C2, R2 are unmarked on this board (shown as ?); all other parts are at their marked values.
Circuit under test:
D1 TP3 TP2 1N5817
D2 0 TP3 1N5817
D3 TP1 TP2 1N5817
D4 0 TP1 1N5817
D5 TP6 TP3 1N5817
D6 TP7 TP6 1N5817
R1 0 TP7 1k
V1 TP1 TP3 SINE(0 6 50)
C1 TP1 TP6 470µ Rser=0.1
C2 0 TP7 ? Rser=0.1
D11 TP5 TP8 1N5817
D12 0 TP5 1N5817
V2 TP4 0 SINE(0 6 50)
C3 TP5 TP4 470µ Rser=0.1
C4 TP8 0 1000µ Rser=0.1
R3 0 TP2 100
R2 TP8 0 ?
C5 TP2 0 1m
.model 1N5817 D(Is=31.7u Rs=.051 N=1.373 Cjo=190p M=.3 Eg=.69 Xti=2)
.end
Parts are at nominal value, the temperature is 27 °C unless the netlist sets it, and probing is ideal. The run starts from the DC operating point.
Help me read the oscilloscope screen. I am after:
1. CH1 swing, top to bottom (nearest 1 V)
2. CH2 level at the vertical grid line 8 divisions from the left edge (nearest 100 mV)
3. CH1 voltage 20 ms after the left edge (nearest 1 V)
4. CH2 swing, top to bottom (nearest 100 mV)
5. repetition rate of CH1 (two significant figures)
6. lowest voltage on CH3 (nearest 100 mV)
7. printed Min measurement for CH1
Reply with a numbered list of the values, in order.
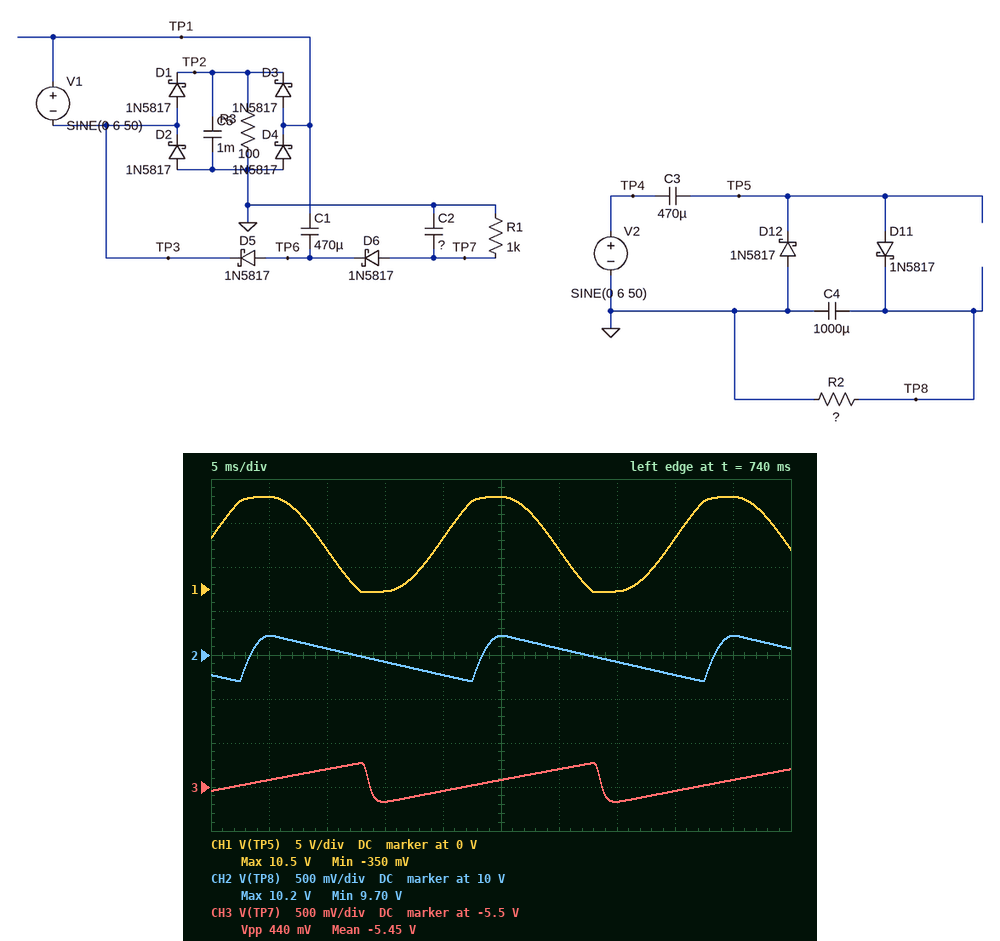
1. 11 V
2. 9.8 V
3. 6 V
4. 500 mV
5. 50 Hz
6. -5.7 V
7. -350 mV
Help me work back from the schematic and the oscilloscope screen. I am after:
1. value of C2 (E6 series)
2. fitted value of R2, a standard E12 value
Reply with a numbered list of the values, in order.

1. 220 µF
2. 330 Ω
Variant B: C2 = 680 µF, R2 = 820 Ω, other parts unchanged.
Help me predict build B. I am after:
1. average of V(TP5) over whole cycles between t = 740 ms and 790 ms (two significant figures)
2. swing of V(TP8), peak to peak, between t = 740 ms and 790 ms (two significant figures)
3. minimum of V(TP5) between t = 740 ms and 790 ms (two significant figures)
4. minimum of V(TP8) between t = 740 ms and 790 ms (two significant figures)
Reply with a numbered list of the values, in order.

1. 5.5 V
2. 240 mV
3. -340 mV
4. 11 V
